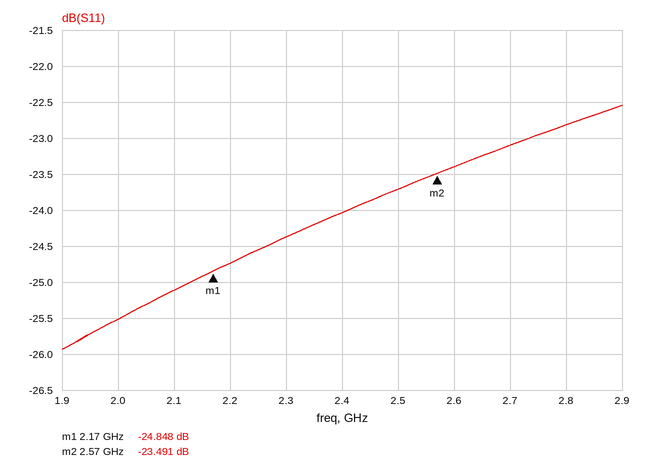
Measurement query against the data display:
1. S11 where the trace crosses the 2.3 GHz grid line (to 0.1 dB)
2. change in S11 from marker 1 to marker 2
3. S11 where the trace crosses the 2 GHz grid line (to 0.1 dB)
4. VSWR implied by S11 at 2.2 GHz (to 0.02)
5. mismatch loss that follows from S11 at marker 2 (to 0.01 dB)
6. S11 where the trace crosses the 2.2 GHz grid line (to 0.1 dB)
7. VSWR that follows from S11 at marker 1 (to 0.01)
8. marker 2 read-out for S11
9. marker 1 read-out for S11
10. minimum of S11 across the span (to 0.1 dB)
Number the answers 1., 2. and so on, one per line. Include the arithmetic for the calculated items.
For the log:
1. -24.4 dB
2. -23.491 − (-24.848) = 1.357 dB
3. -25.5 dB
4. |Γ| = 10^(-24.7/20) = 0.0582; VSWR = (1 + 0.0582)/(1 − 0.0582) ≈ 1.12
5. −10 log10(1 − 10^(-23.491/10)) ≈ 0.02 dB
6. -24.7 dB
7. (1 + 0.0572)/(1 − 0.0572) ≈ 1.12
8. -23.491 dB
9. -24.848 dB
10. -25.9 dB
